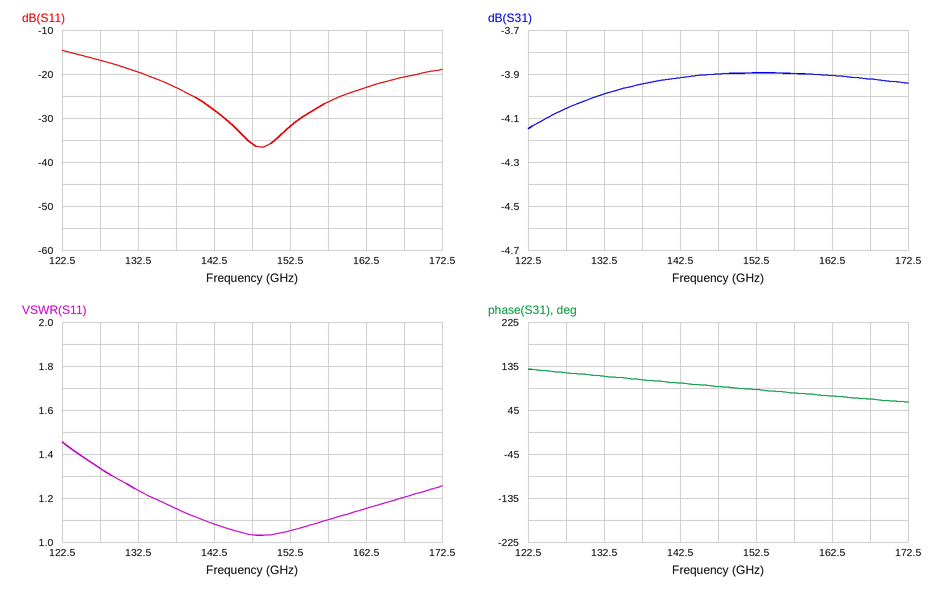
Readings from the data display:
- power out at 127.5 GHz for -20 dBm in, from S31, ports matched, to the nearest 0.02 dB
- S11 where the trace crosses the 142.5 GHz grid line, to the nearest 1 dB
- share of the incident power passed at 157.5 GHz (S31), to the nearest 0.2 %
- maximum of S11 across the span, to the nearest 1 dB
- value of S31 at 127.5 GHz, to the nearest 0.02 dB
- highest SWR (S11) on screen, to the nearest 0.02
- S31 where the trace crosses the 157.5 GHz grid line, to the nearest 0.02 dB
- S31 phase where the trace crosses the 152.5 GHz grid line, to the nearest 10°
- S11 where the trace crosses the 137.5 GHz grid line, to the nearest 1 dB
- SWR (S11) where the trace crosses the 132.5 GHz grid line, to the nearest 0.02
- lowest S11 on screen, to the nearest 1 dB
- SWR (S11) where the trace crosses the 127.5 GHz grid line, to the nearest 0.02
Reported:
-24.06 dBm
-28 dB
40.8 %
-15 dB
-4.06 dB
1.46
-3.90 dB
90°
-23 dB
1.24
-37 dB
1.34
